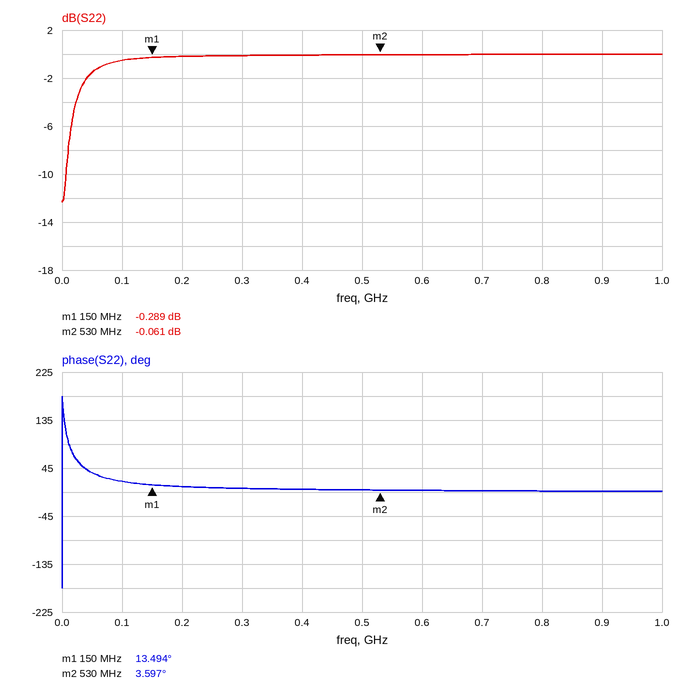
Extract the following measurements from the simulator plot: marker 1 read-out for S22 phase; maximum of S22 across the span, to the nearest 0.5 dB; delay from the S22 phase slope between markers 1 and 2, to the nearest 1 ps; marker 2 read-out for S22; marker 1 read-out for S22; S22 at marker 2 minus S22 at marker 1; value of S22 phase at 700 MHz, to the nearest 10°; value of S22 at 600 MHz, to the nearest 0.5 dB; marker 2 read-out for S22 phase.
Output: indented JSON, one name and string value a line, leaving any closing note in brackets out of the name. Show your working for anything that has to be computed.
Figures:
{
  "marker 1 read-out for S22 phase": "13.494°",
  "maximum of S22 across the span, to the nearest 0.5 dB": "0.0 dB",
  "delay from the S22 phase slope between markers 1 and 2, to the nearest 1 ps": "−(3.597° − (13.494°))/(360° × 380 MHz) ≈ 72 ps",
  "marker 2 read-out for S22": "-0.061 dB",
  "marker 1 read-out for S22": "-0.289 dB",
  "S22 at marker 2 minus S22 at marker 1": "-0.061 − (-0.289) = 0.228 dB",
  "value of S22 phase at 700 MHz, to the nearest 10°": "0°",
  "value of S22 at 600 MHz, to the nearest 0.5 dB": "0.0 dB",
  "marker 2 read-out for S22 phase": "3.597°"
}
